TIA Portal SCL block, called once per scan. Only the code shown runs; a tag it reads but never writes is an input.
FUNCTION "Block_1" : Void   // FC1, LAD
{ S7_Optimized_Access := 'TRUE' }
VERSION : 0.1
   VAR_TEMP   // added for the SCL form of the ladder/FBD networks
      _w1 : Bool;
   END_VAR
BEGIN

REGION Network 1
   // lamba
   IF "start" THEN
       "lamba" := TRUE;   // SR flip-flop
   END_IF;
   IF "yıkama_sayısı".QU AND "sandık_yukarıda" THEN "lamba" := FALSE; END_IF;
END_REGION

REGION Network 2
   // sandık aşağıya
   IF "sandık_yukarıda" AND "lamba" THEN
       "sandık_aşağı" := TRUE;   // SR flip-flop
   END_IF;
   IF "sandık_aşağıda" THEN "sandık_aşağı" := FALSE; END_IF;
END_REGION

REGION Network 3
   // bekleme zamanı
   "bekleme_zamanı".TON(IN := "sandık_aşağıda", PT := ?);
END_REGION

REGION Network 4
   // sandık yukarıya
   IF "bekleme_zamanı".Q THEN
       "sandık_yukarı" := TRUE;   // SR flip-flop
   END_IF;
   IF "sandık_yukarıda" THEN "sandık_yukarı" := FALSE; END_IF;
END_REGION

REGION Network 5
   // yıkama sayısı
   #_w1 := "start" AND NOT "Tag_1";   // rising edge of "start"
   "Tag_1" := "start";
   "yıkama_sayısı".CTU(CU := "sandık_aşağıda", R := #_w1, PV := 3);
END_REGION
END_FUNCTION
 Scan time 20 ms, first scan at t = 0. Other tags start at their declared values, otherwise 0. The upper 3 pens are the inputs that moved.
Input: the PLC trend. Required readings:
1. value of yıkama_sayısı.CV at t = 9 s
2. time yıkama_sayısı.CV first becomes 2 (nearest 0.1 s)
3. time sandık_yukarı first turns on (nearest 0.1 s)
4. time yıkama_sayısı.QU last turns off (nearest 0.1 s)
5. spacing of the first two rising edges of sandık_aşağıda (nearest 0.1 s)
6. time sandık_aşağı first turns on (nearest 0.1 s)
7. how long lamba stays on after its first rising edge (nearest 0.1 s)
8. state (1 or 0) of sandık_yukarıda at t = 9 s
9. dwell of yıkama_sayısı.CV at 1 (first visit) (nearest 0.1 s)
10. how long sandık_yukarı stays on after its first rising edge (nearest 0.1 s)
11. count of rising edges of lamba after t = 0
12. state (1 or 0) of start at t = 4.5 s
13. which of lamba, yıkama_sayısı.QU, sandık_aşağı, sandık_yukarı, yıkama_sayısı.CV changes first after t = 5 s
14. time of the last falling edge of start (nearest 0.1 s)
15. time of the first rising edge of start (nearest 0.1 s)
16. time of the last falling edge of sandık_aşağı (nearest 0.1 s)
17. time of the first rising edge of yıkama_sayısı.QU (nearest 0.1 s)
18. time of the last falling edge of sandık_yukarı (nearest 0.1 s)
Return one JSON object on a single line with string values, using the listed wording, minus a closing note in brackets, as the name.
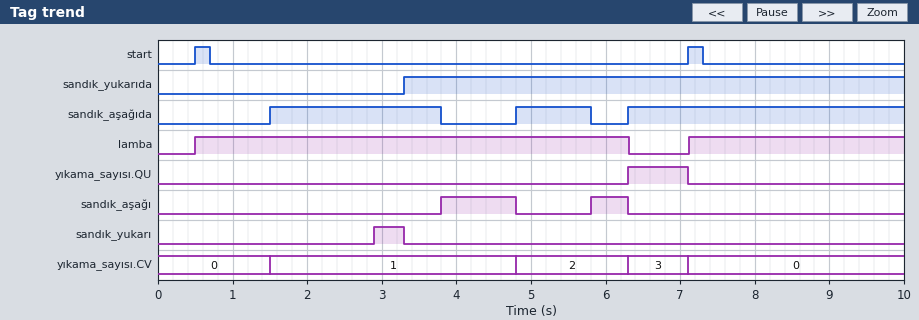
{"value of yıkama_sayısı.CV at t = 9 s": "0", "time yıkama_sayısı.CV first becomes 2": "4.8 s", "time sandık_yukarı first turns on": "2.9 s", "time yıkama_sayısı.QU last turns off": "7.1 s", "spacing of the first two rising edges of sandık_aşağıda": "3.3 s", "time sandık_aşağı first turns on": "3.8 s", "how long lamba stays on after its first rising edge": "5.8 s", "state (1 or 0) of sandık_yukarıda at t = 9 s": "1", "dwell of yıkama_sayısı.CV at 1 (first visit)": "3.3 s", "how long sandık_yukarı stays on after its first rising edge": "0.4 s", "count of rising edges of lamba after t = 0": "2", "state (1 or 0) of start at t = 4.5 s": "0", "which of lamba, yıkama_sayısı.QU, sandık_aşağı, sandık_yukarı, yıkama_sayısı.CV changes first after t = 5 s": "sandık_aşağı", "time of the last falling edge of start": "7.3 s", "time of the first rising edge of start": "0.5 s", "time of the last falling edge of sandık_aşağı": "6.3 s", "time of the first rising edge of yıkama_sayısı.QU": "6.3 s", "time of the last falling edge of sandık_yukarı": "3.3 s"}
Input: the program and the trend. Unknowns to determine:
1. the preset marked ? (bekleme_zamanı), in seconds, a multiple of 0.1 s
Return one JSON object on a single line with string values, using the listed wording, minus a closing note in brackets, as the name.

{"the preset marked ? (bekleme_zamanı), in seconds, a multiple of 0.1 s": "1.4 s"}
